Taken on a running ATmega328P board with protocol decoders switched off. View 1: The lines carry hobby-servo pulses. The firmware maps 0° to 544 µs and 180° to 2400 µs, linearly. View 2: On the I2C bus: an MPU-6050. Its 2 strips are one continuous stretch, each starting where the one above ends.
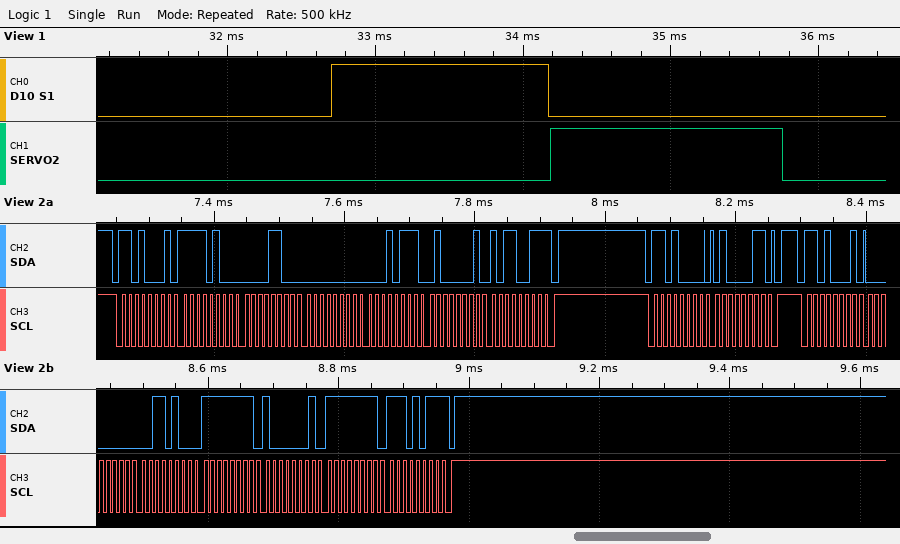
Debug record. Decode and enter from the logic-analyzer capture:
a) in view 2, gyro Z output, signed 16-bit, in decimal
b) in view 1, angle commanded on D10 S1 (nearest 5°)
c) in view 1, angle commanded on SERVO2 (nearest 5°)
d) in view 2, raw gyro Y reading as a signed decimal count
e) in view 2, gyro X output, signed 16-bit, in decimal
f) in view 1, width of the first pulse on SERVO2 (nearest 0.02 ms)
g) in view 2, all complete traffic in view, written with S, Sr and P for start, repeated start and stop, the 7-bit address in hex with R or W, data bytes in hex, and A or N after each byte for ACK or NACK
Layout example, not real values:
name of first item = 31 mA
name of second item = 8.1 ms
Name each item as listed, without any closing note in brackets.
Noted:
in view 2, gyro Z output, signed 16-bit, in decimal = -21
in view 1, angle commanded on D10 S1 = 90°
in view 1, angle commanded on SERVO2 = 100°
in view 2, raw gyro Y reading as a signed decimal count = -127
in view 2, gyro X output, signed 16-bit, in decimal = 52
in view 1, width of the first pulse on SERVO2 = 1.58 ms
in view 2, all complete traffic in view, written with S, Sr and P for start, repeated start and stop, the 7-bit address in hex with R or W, data bytes in hex, and A or N after each byte for ACK or NACK = S 68R A F4 A 0C A 00 A 17 A 41 A B3 N P S 68W A 43 A P S 68R A 00 A 34 A FF A 81 A FF A EB N P
